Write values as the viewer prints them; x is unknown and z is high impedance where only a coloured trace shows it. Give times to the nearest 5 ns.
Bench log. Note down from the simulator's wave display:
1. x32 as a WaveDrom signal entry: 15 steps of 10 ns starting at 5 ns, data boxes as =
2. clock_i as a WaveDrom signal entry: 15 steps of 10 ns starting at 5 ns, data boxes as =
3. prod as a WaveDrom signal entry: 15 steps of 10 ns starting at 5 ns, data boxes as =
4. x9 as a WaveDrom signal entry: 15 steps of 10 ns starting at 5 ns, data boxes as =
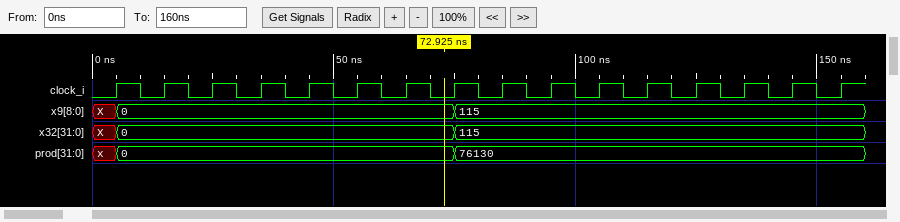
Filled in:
{name: 'x32', wave: '=......=.......', data: '0 115'}
{name: 'clock_i', wave: 'p..............'}
{name: 'prod', wave: '=......=.......', data: '0 76130'}
{name: 'x9', wave: '=......=.......', data: '0 115'}
